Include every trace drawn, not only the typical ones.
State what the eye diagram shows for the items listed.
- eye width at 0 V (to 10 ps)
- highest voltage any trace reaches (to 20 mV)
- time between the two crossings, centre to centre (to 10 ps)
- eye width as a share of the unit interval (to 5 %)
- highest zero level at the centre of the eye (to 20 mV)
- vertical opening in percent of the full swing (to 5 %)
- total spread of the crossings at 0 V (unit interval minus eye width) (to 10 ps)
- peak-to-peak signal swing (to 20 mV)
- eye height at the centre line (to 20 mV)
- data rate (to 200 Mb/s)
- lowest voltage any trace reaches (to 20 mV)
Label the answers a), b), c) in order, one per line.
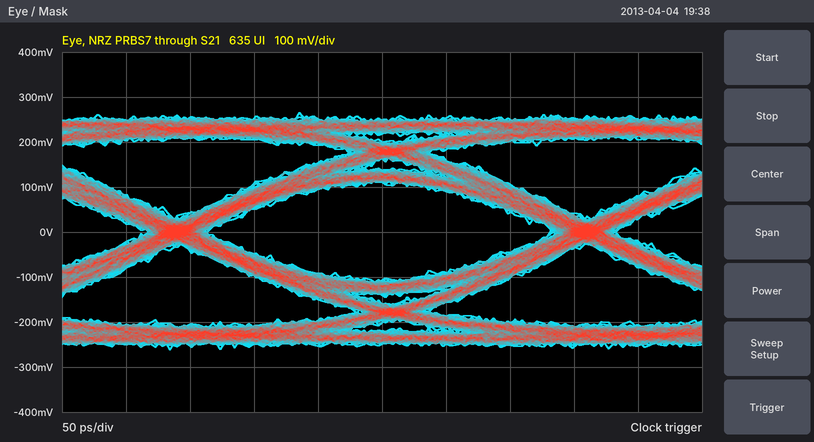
a) 270 ps
b) 260 mV
c) 320 ps
d) 85 %
e) -100 mV
f) 40 %
g) 50 ps
h) 520 mV
i) 220 mV
j) 3.2 Gb/s
k) -260 mV
